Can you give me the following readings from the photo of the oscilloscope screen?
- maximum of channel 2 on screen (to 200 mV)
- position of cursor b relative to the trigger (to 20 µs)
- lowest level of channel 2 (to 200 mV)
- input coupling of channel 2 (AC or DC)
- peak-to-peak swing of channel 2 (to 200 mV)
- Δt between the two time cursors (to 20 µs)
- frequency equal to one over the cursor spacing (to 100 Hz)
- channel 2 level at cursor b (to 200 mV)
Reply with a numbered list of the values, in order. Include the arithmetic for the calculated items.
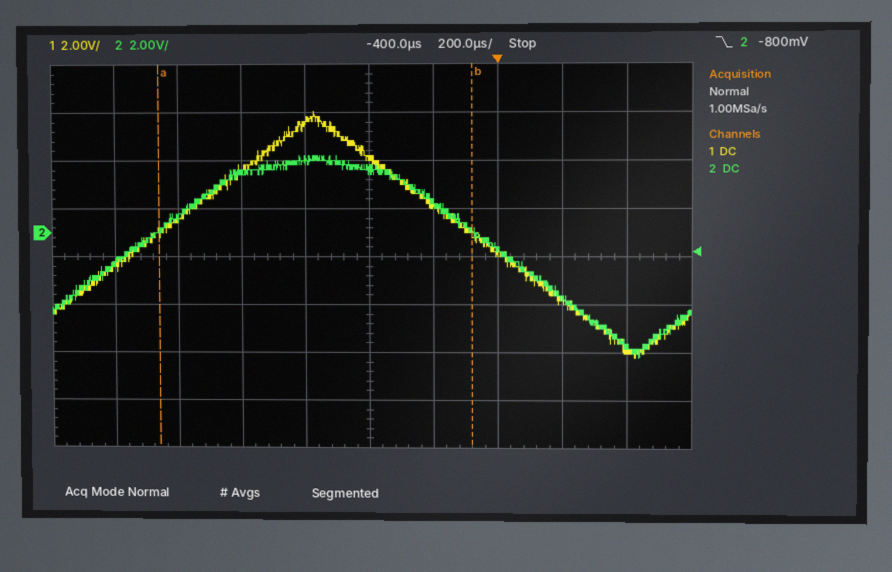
1. 3.2 V
2. -80 µs
3. -5.2 V
4. DC
5. 3.2 V − (-5.2 V) = 8.4 V
6. 980 µs
7. 1 / 980 µs ≈ 1.0 kHz
8. 0.0 V
